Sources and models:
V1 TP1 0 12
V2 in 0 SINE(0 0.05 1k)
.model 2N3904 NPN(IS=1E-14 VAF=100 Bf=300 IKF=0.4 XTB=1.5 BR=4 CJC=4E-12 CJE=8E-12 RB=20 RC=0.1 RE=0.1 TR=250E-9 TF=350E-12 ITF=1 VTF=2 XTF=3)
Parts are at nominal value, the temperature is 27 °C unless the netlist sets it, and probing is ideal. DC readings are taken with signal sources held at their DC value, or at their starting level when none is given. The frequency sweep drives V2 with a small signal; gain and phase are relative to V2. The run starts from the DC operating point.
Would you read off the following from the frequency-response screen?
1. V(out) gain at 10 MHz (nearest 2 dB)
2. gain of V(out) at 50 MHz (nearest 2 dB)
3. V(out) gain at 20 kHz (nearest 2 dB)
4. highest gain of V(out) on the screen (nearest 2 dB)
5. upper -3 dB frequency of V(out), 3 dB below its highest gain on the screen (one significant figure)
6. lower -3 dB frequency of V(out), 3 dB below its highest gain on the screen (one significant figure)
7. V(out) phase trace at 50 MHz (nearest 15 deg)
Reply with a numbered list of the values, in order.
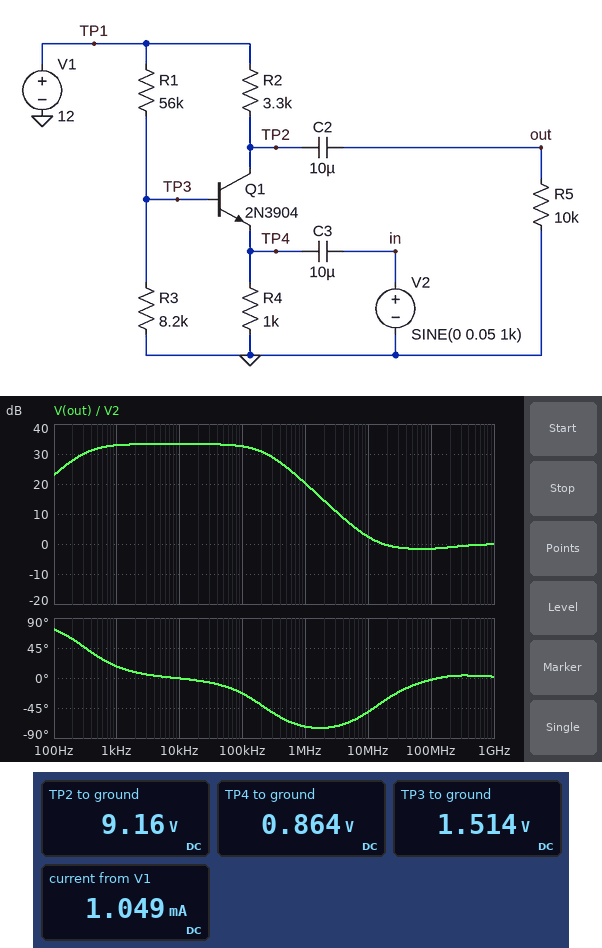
1. 2 dB
2. -2 dB
3. 34 dB
4. 34 dB
5. 200 kHz
6. 300 Hz
7. -15 deg
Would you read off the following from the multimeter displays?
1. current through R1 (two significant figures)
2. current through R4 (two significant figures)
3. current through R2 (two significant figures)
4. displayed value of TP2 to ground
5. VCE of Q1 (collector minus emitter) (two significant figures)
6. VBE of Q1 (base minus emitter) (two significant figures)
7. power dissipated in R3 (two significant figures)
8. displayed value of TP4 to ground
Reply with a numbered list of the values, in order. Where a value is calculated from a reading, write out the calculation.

1. (12 V - 1.514 V) / 56 kΩ = 190 µA
2. (864 mV) / 1 kΩ = 860 µA
3. (12 V - 9.16 V) / 3.3 kΩ = 860 µA
4. 9.16 V
5. 9.16 V - 864 mV = 8.3 V
6. 1.514 V - 864 mV = 650 mV
7. (1.514 V)^2 / 8.2 kΩ = 280 µW
8. 0.864 V
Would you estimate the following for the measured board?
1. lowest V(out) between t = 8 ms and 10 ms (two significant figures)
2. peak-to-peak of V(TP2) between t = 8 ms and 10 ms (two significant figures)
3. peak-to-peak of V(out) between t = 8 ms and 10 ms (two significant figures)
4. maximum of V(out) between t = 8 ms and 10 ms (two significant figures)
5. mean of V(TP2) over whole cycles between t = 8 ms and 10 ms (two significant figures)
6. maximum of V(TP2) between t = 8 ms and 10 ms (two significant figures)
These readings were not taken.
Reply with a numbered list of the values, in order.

1. -2.3 V
2. 4.0 V
3. 4.0 V
4. 1.7 V
5. 9.1 V
6. 11 V
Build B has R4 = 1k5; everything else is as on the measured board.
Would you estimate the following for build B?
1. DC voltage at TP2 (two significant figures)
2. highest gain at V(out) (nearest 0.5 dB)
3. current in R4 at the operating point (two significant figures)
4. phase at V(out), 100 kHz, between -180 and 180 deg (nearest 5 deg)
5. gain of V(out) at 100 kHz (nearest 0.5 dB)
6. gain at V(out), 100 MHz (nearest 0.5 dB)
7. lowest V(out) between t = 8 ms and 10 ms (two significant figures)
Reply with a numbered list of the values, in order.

1. 10 V
2. 31.5 dB
3. 590 µA
4. -20 deg
5. 31.0 dB
6. -2.0 dB
7. -1.9 V
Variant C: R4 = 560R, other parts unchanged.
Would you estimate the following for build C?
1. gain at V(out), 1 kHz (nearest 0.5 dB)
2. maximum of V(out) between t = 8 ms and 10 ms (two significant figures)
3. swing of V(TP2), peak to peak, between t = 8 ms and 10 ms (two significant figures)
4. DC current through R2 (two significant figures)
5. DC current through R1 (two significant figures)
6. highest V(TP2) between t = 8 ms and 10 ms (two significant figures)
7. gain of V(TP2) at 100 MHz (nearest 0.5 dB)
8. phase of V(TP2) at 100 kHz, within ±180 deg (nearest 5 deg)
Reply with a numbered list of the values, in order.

1. 35.0 dB
2. 2.4 V
3. 5.2 V
4. 1.5 mA
5. 190 µA
6. 9.5 V
7. -1.0 dB
8. -30 deg
